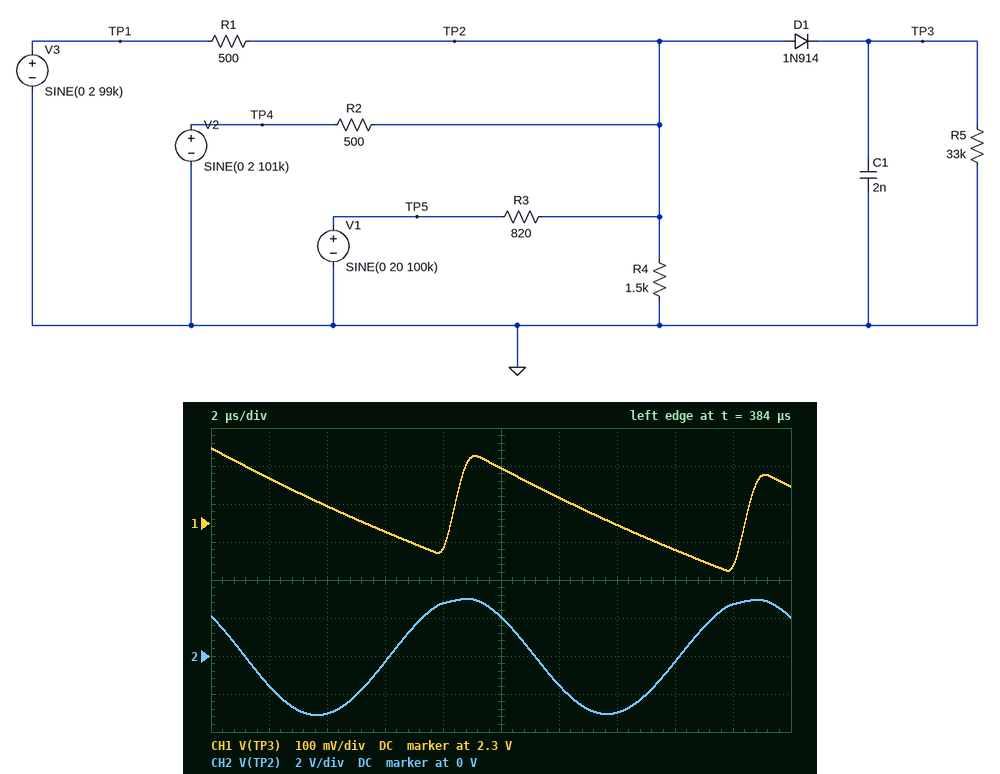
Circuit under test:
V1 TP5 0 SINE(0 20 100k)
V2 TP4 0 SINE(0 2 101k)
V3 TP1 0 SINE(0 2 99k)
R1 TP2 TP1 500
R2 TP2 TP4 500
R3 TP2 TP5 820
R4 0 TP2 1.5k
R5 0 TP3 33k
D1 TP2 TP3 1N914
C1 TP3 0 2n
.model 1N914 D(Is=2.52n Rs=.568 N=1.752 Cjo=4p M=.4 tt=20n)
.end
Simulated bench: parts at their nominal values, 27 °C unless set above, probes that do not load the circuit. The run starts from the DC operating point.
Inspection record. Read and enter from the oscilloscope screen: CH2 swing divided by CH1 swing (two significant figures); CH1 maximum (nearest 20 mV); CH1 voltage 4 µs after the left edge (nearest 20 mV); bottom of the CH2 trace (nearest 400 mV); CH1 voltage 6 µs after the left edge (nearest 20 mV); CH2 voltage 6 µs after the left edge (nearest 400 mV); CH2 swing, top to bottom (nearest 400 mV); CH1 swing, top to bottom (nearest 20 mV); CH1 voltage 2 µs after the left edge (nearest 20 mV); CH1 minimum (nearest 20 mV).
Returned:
19
2.50 V
2.34 V
-3.2 V
2.28 V
-400 mV
6.0 V
320 mV
2.42 V
2.18 V
